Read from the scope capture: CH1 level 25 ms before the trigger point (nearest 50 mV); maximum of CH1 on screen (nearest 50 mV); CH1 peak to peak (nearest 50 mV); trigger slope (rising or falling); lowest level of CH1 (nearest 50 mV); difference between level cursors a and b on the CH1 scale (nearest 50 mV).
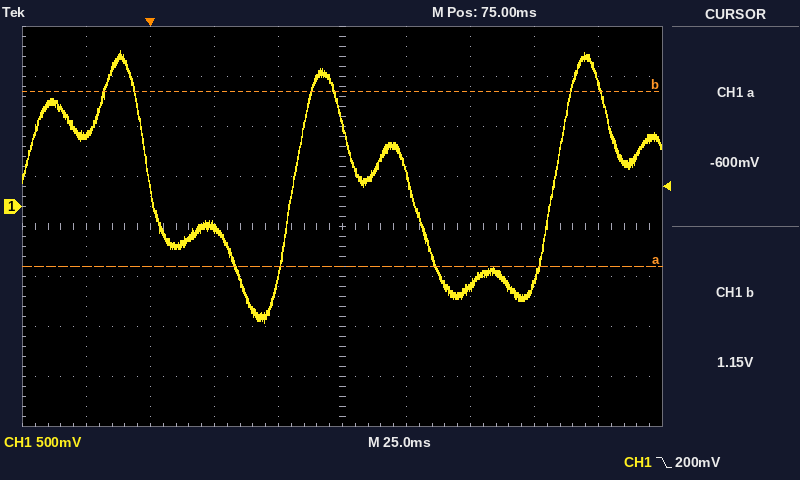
700 mV
1.55 V
2.70 V
falling
-1.15 V
1.75 V
